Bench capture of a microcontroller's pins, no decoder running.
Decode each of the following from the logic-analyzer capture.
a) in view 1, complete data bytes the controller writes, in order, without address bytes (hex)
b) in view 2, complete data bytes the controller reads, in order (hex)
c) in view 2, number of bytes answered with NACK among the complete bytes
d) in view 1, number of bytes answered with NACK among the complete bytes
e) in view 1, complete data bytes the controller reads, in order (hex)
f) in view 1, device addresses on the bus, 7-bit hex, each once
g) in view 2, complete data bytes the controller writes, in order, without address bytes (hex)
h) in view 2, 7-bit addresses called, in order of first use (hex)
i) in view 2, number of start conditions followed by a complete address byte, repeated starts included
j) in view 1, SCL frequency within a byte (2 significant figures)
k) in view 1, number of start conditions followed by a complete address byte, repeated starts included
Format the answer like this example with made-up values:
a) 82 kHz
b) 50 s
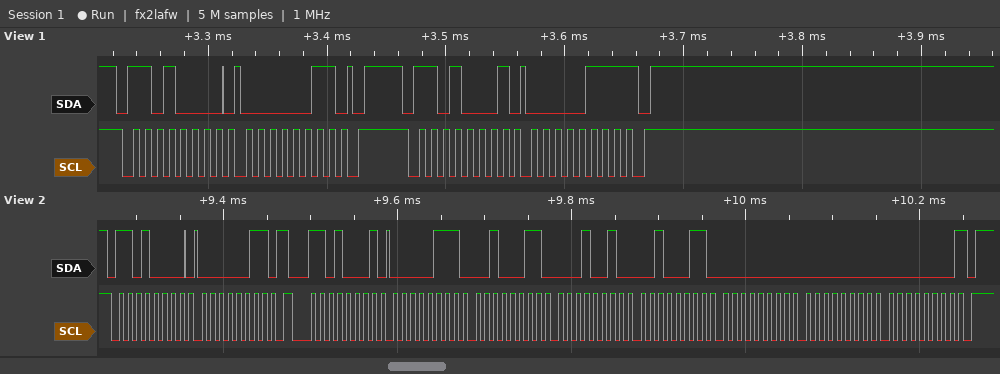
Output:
a) 03
b) 07 23 12 23 00 00 00
c) 1
d) 1
e) 07
f) 0x68
g) 03
h) 0x68
i) 2
j) 100 kHz
k) 2
